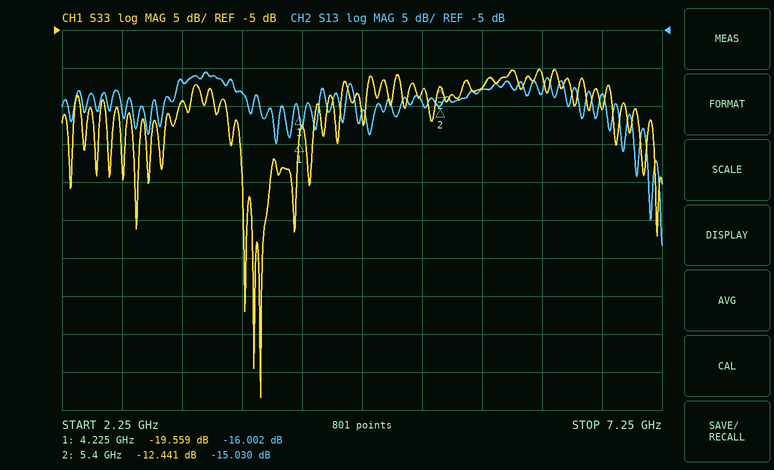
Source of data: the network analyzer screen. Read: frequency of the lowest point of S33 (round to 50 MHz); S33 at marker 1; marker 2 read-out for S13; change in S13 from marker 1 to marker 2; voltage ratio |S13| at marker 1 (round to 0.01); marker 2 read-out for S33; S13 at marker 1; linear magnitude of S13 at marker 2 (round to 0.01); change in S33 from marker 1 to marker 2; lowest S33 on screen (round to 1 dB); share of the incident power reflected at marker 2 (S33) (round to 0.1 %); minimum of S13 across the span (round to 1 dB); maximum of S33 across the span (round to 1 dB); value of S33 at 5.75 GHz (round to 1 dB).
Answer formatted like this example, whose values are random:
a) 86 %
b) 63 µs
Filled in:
a) 3.90 GHz
b) -19.559 dB
c) -15.030 dB
d) 0.972 dB
e) 0.16
f) -12.441 dB
g) -16.002 dB
h) 0.18
i) 7.118 dB
j) -53 dB
k) 5.7 %
l) -33 dB
m) -10 dB
n) -13 dB
